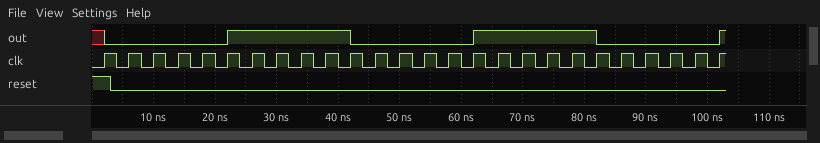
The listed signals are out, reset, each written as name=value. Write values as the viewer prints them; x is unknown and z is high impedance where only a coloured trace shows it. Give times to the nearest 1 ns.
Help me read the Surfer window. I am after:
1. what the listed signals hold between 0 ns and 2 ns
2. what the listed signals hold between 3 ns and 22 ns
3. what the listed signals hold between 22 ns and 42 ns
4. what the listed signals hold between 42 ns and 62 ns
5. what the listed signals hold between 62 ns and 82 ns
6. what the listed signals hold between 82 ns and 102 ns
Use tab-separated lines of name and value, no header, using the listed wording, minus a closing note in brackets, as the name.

what the listed signals hold between 0 ns and 2 ns	out=x, reset=1
what the listed signals hold between 3 ns and 22 ns	out=0, reset=0
what the listed signals hold between 22 ns and 42 ns	out=1, reset=0
what the listed signals hold between 42 ns and 62 ns	out=0, reset=0
what the listed signals hold between 62 ns and 82 ns	out=1, reset=0
what the listed signals hold between 82 ns and 102 ns	out=0, reset=0
